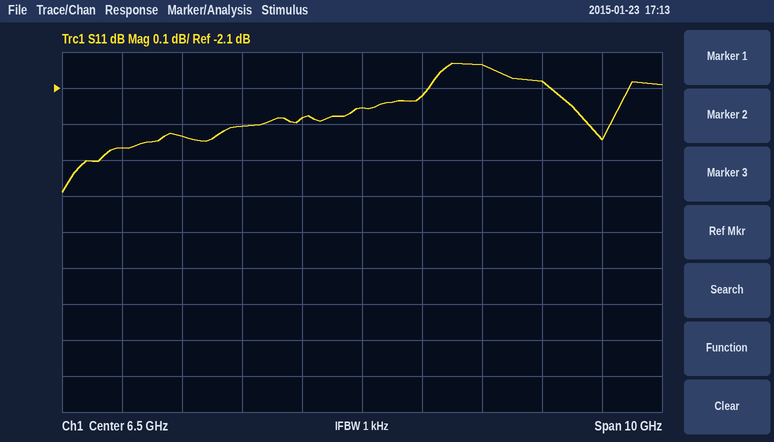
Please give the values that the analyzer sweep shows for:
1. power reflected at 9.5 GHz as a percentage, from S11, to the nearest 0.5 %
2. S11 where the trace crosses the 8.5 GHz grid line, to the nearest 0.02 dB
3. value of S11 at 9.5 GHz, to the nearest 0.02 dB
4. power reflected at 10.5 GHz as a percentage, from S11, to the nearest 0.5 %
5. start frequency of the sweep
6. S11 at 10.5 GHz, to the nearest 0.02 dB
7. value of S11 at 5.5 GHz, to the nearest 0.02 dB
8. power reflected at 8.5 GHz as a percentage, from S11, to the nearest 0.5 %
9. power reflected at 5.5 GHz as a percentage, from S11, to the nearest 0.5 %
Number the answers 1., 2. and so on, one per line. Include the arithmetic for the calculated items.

1. 10^(-2.08/10) ≈ 61.9 %, so 62.0 % to the nearest 0.5 %
2. -2.04 dB
3. -2.08 dB
4. 10^(-2.24/10) ≈ 59.7 %, so 59.5 % to the nearest 0.5 %
5. 1.5 GHz
6. -2.24 dB
7. -2.18 dB
8. 10^(-2.04/10) ≈ 62.5 %
9. 10^(-2.18/10) ≈ 60.5 %
